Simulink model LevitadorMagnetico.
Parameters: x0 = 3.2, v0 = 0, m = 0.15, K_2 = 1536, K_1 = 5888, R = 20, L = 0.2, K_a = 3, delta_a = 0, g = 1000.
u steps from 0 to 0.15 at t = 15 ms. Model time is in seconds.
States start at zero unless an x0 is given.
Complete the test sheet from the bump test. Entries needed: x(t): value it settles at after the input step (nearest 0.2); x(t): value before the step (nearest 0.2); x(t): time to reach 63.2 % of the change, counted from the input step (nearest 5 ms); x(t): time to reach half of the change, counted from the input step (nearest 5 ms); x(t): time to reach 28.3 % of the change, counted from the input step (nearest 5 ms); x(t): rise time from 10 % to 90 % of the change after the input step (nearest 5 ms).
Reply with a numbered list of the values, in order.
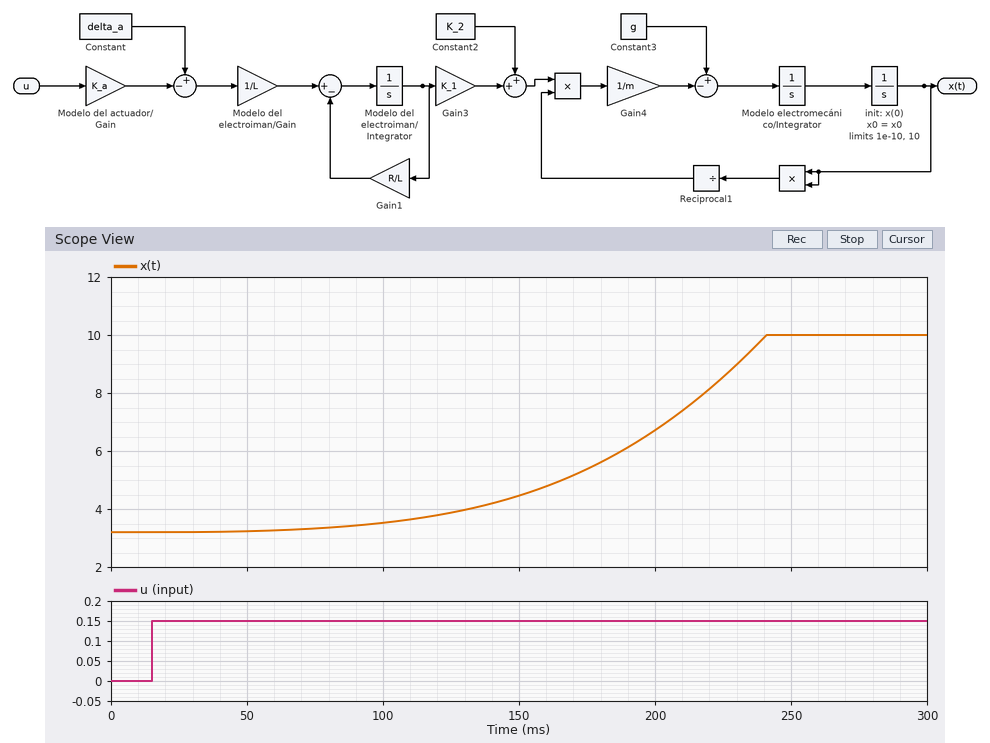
1. 10.0
2. 3.2
3. 195 ms
4. 185 ms
5. 155 ms
6. 110 ms
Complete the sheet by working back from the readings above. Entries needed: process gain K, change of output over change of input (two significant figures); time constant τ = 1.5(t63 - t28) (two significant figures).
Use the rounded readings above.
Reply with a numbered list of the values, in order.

1. 45
2. 60 ms
